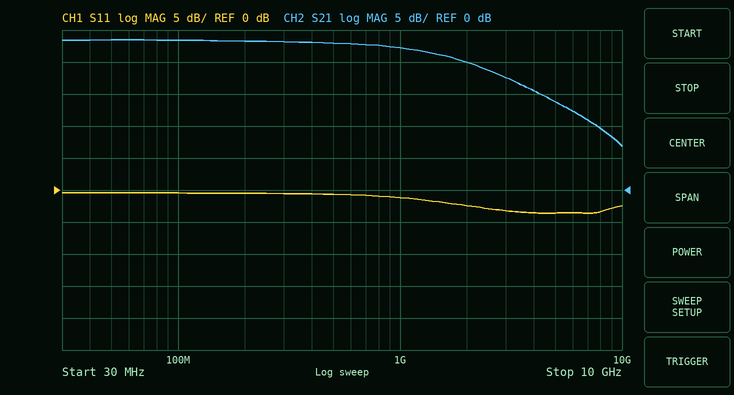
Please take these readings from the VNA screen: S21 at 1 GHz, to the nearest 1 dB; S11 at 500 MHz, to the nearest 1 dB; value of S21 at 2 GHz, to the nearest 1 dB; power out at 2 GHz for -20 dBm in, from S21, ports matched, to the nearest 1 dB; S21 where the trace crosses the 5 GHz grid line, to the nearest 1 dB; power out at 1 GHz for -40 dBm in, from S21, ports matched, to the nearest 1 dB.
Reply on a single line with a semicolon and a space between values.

22 dB; -1 dB; 20 dB; 0 dBm; 14 dB; -18 dBm
